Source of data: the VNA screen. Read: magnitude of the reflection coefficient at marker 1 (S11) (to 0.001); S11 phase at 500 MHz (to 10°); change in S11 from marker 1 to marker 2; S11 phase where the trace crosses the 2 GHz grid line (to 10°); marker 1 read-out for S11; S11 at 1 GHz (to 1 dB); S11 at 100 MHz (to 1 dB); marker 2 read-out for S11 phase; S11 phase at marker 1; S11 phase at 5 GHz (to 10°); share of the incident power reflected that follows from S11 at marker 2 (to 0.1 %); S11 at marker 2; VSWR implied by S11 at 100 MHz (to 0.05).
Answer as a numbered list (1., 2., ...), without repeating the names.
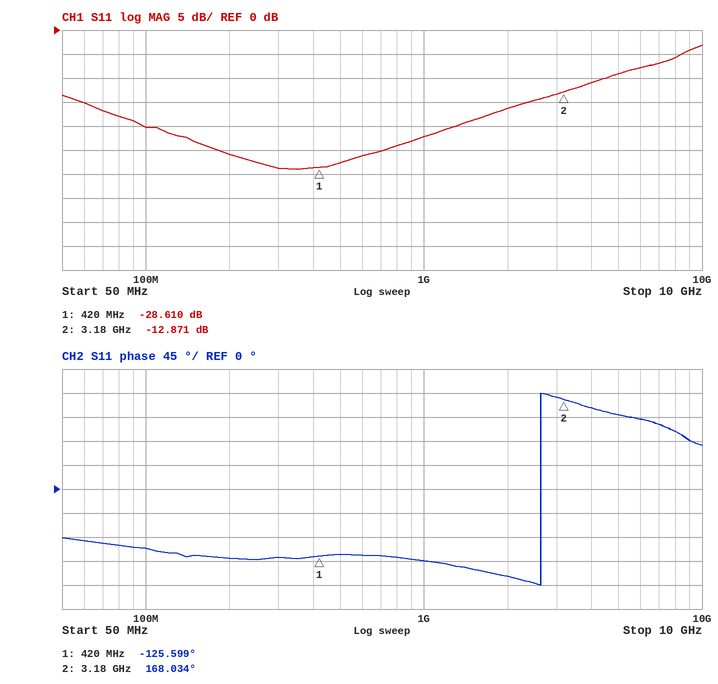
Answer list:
1. 0.037
2. -120°
3. 15.739 dB
4. -160°
5. -28.610 dB
6. -22 dB
7. -20 dB
8. 168.034°
9. -125.599°
10. 140°
11. 5.2 %
12. -12.871 dB
13. 1.20
